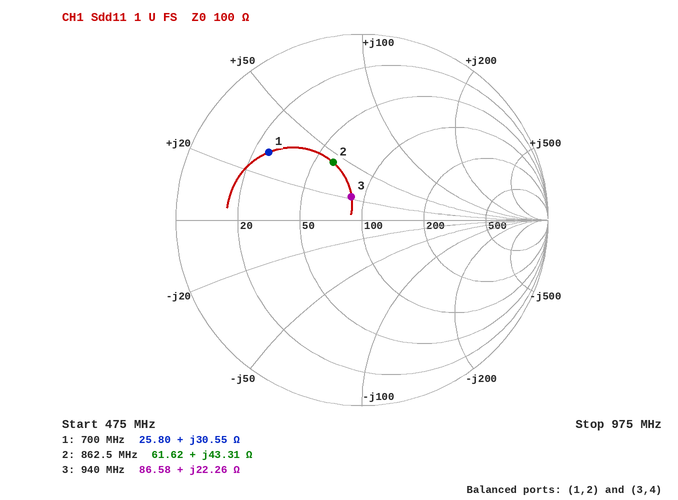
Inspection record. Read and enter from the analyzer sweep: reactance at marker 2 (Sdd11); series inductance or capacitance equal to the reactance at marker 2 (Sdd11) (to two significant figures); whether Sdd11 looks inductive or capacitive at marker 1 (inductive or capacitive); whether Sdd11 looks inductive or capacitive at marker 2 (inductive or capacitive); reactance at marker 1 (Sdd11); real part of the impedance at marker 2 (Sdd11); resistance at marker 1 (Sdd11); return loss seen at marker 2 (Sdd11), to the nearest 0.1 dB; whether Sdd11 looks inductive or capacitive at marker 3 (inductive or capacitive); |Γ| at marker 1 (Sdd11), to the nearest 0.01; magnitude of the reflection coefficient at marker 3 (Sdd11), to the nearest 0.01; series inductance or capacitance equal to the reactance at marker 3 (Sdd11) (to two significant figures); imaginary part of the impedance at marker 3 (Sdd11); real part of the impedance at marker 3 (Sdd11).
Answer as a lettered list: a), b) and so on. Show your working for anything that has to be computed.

a) +43.31 Ω
b) L = 43.31 Ω/(2π × 862.5 MHz) ≈ 8.0 nH
c) inductive
d) inductive
e) +30.55 Ω
f) 61.62 Ω
g) 25.80 Ω
h) 9.2 dB
i) inductive
j) 0.62
k) 0.14
l) L = 22.26 Ω/(2π × 940 MHz) ≈ 3.8 nH
m) +22.26 Ω
n) 86.58 Ω
